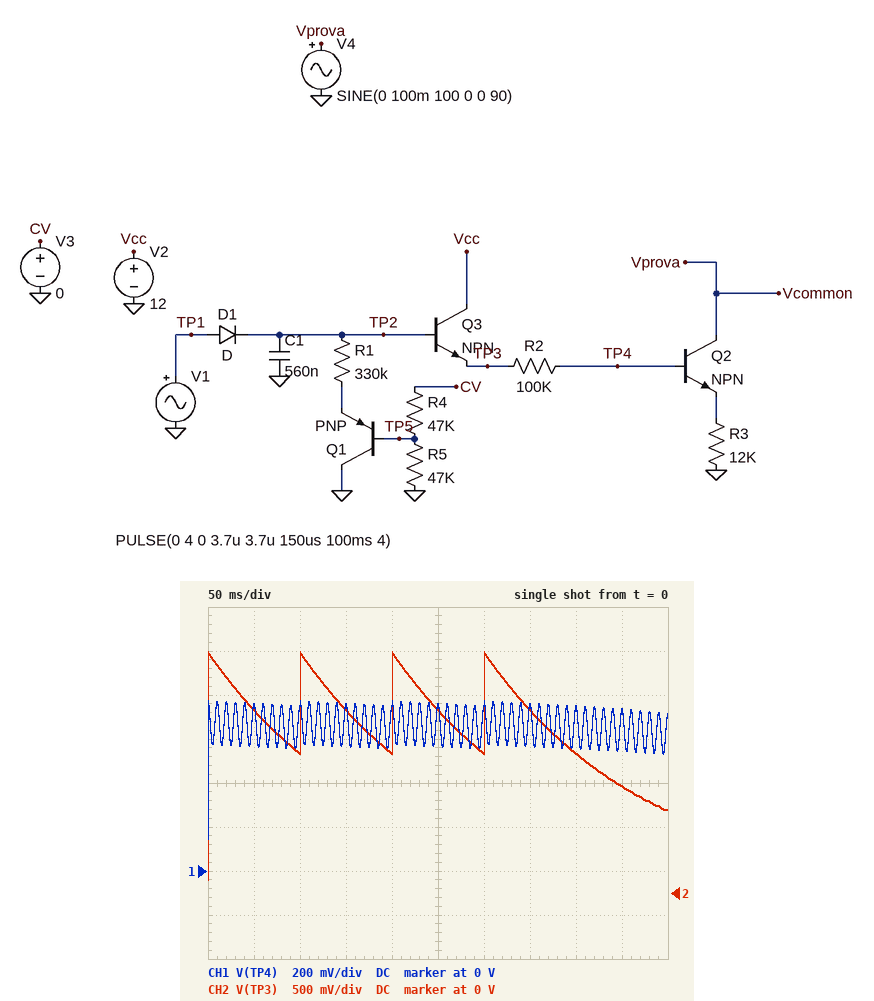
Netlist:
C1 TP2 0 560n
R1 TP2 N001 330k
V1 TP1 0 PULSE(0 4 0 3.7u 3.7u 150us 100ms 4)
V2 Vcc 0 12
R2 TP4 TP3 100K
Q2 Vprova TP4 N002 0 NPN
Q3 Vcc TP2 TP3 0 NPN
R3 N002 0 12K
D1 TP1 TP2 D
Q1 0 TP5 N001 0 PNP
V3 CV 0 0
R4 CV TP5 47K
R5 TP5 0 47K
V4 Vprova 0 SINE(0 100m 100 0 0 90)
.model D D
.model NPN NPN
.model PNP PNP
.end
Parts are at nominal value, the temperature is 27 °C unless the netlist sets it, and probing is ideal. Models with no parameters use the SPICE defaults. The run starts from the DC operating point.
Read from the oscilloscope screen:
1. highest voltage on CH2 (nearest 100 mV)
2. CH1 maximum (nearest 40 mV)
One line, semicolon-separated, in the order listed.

2.7 V; 760 mV
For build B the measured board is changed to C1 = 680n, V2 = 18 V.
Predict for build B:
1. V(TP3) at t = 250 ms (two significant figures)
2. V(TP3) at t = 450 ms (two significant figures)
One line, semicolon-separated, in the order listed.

2.2 V; 1.4 V
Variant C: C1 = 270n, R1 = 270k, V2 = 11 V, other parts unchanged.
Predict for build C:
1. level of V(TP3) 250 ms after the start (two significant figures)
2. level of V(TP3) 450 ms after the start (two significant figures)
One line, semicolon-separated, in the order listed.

1.4 V; 530 mV
